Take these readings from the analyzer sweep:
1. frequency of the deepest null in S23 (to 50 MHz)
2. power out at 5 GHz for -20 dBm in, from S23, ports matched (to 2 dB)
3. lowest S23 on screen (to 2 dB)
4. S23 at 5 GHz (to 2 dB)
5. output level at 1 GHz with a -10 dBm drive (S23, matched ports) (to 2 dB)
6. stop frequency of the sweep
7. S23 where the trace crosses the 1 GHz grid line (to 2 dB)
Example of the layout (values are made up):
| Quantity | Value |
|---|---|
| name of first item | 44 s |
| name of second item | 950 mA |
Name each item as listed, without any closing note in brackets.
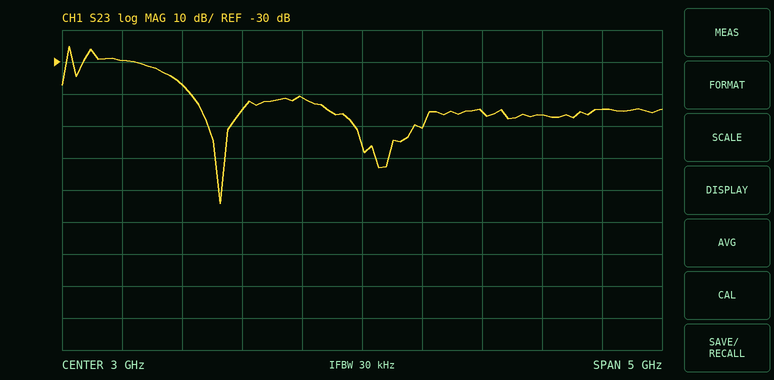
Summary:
| Quantity | Value |
|---|---|
| frequency of the deepest null in S23 | 1.80 GHz |
| power out at 5 GHz for -20 dBm in, from S23, ports matched | -64 dBm |
| lowest S23 on screen | -74 dB |
| S23 at 5 GHz | -44 dB |
| output level at 1 GHz with a -10 dBm drive (S23, matched ports) | -40 dBm |
| stop frequency of the sweep | 5.5 GHz |
| S23 where the trace crosses the 1 GHz grid line | -30 dB |
